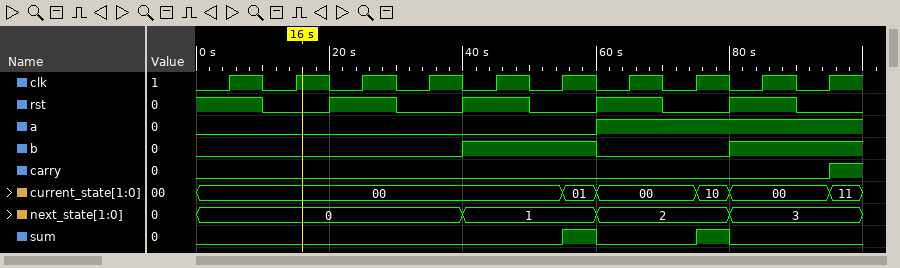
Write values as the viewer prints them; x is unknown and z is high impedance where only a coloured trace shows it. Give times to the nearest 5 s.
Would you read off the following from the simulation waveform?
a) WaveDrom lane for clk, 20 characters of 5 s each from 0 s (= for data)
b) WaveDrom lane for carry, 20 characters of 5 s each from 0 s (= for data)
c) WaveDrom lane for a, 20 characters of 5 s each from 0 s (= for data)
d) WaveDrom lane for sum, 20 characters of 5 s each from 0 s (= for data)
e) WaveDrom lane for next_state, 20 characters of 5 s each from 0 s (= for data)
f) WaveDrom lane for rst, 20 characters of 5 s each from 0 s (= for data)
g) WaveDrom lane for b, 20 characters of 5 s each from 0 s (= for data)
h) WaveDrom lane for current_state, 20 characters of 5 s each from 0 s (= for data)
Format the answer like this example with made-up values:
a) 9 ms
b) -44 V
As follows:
a) {name: 'clk', wave: '01010101010101010101'}
b) {name: 'carry', wave: '0..................1'}
c) {name: 'a', wave: '0...........1.......'}
d) {name: 'sum', wave: '0..........10..10...'}
e) {name: 'next_state', wave: '=.......=...=...=...', data: '0 1 2 3'}
f) {name: 'rst', wave: '1.0.1.0.1.0.1.0.1.0.'}
g) {name: 'b', wave: '0.......1...0...1...'}
h) {name: 'current_state', wave: '=..........==..==..=', data: '00 01 00 10 00 11'}
